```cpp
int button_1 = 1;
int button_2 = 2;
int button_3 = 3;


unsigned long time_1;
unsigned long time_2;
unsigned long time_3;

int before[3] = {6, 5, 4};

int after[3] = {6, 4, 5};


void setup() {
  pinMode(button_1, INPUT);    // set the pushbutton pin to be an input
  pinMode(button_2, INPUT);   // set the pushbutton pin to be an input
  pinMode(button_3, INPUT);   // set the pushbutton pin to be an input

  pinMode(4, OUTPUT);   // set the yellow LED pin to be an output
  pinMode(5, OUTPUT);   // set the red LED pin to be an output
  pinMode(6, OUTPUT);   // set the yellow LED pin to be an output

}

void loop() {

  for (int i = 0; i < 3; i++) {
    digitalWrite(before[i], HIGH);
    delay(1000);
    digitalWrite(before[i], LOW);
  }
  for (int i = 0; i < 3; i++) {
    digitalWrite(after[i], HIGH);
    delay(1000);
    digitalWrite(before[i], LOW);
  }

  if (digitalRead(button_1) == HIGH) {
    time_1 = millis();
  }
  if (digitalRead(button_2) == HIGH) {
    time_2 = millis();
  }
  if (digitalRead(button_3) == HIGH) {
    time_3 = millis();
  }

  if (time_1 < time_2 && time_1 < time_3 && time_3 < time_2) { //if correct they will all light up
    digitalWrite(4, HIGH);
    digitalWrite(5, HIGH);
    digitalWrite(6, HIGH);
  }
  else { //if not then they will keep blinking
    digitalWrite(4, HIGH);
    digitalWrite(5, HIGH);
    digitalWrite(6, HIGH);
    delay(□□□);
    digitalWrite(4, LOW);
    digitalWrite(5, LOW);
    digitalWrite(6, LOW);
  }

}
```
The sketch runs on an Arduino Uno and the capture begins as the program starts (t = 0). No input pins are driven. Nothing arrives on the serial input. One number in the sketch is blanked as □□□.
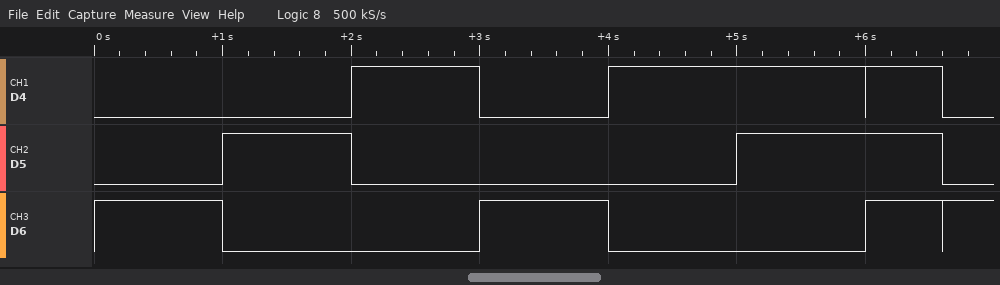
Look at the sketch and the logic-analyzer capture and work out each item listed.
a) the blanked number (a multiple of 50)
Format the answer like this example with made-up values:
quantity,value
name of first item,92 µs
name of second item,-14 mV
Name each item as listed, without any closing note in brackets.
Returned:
quantity,value
the blanked number,600
